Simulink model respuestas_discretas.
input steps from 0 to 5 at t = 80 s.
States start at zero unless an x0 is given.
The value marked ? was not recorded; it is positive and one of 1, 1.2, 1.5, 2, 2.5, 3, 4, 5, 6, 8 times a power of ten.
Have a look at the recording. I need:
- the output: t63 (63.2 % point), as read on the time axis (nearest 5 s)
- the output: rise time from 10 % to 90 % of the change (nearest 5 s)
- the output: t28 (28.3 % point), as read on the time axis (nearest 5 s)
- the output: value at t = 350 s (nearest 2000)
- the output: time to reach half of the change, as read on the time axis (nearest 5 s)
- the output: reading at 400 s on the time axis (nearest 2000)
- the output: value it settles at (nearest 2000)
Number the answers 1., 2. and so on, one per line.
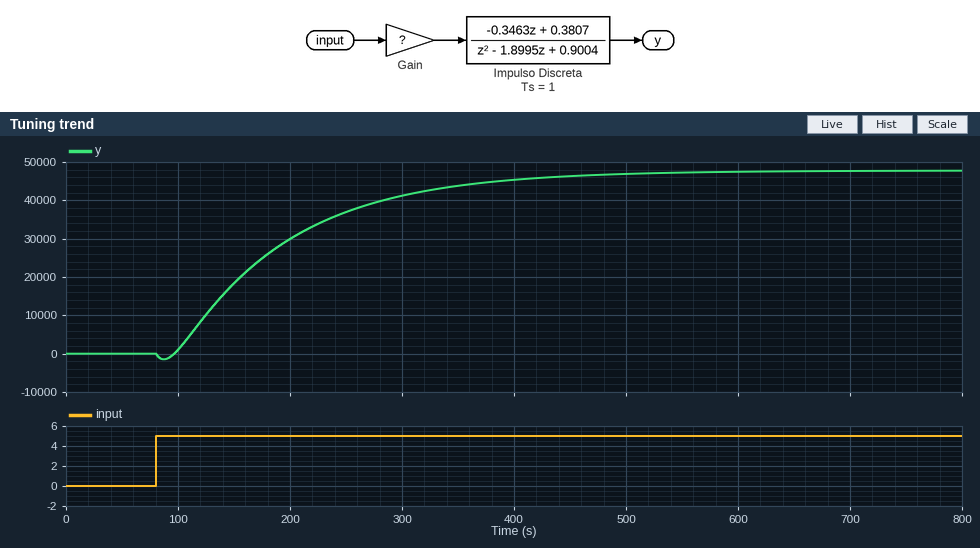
1. 200 s
2. 220 s
3. 135 s
4. 44000
5. 170 s
6. 46000
7. 48000
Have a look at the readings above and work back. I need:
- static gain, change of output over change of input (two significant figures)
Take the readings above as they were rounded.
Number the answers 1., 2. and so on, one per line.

1. 9600
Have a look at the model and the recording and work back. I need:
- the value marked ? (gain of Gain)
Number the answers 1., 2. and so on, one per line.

1. 250
